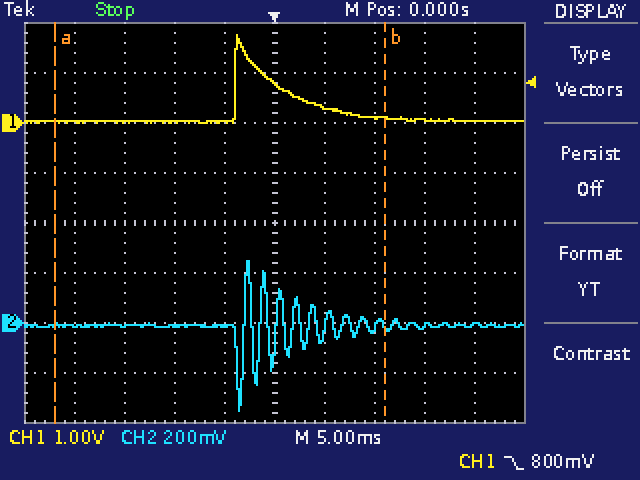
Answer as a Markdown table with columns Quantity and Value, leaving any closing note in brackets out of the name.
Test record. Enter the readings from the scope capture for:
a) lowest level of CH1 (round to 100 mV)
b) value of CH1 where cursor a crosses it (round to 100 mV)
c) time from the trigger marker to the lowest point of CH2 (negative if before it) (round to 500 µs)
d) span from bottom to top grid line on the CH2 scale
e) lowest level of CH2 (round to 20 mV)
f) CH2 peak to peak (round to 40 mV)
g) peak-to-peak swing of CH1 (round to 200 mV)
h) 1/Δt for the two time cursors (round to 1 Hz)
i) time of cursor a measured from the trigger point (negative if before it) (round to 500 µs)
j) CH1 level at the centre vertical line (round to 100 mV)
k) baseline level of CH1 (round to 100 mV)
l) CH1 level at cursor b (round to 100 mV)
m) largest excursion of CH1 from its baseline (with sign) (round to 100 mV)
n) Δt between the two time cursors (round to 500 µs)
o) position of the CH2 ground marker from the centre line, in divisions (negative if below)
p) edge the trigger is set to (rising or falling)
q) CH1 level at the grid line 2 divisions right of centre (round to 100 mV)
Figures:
| Quantity | Value |
|---|---|
| lowest level of CH1 | 0.0 V |
| value of CH1 where cursor a crosses it | 0.0 V |
| time from the trigger marker to the lowest point of CH2 (negative if before it) | -3.5 ms |
| span from bottom to top grid line on the CH2 scale | 1.6 V |
| lowest level of CH2 | -360 mV |
| CH2 peak to peak | 600 mV |
| peak-to-peak swing of CH1 | 1.8 V |
| 1/Δt for the two time cursors | 30 Hz |
| time of cursor a measured from the trigger point (negative if before it) | -22.0 ms |
| CH1 level at the centre vertical line | 800 mV |
| baseline level of CH1 | 0.0 V |
| CH1 level at cursor b | 100 mV |
| largest excursion of CH1 from its baseline (with sign) | +1.7 V |
| Δt between the two time cursors | 33.0 ms |
| position of the CH2 ground marker from the centre line, in divisions | -2.0 div |
| edge the trigger is set to | falling |
| CH1 level at the grid line 2 divisions right of centre | 100 mV |
